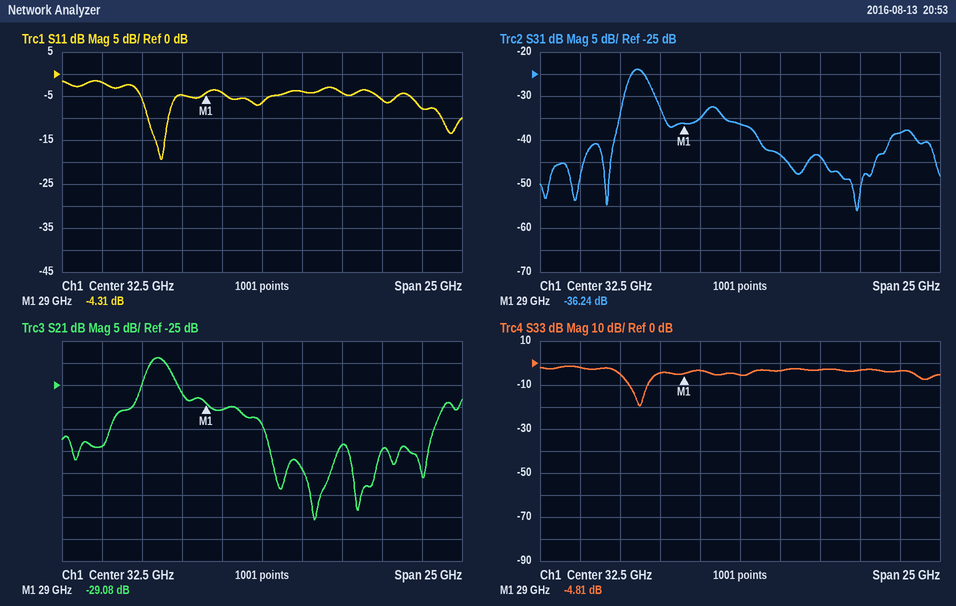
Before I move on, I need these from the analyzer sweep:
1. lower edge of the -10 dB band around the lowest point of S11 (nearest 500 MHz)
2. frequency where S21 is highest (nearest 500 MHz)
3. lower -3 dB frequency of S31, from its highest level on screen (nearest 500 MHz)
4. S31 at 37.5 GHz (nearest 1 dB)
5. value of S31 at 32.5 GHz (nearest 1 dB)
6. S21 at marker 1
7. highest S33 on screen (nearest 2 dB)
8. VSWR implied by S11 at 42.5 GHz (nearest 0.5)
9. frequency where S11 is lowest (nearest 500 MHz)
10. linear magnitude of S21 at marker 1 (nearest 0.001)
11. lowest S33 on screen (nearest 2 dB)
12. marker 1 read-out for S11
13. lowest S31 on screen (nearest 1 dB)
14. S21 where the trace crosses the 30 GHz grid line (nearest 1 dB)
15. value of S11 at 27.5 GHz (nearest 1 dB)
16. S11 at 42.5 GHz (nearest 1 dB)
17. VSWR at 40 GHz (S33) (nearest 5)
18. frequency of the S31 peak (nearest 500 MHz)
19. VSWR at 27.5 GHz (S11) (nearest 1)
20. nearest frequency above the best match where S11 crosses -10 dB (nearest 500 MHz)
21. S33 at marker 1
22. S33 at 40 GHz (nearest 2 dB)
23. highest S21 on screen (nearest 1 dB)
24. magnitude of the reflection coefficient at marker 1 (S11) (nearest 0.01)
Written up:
25.5 GHz
26.0 GHz
25.5 GHz
-44 dB
-36 dB
-29.08 dB
-2 dB
2.5
26.0 GHz
0.035
-20 dB
-4.31 dB
-56 dB
-31 dB
-5 dB
-8 dB
5
26.0 GHz
4
26.5 GHz
-4.81 dB
-4 dB
-19 dB
0.61
